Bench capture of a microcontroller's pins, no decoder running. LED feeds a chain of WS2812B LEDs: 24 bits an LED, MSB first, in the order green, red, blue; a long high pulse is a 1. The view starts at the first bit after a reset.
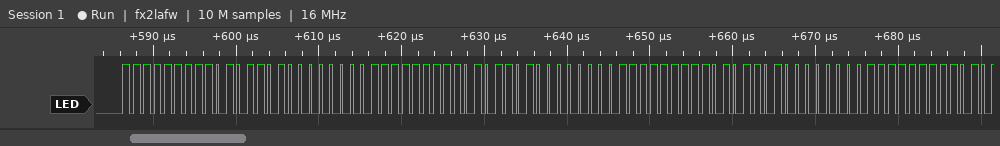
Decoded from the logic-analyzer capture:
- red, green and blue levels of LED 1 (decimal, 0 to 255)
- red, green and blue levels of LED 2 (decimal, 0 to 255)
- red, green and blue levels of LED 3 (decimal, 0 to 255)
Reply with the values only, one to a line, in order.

173, 255, 0
173, 255, 0
173, 255, 0
